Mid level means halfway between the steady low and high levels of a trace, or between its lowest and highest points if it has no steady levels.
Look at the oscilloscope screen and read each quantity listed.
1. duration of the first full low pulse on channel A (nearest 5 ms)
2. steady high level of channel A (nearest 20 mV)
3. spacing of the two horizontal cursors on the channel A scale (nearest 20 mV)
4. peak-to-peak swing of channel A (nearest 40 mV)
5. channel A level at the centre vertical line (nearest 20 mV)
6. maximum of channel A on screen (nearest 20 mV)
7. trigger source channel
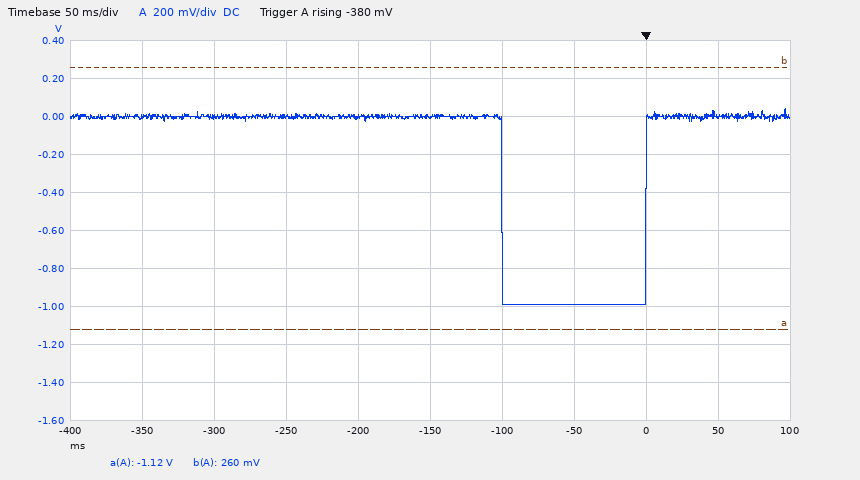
100 ms
0 mV
1.38 V
1.04 V
0 mV
40 mV
channel A
